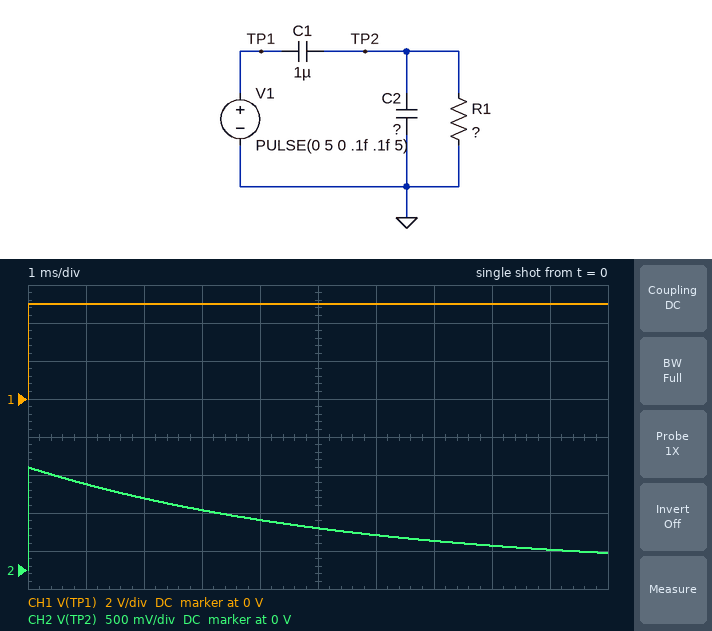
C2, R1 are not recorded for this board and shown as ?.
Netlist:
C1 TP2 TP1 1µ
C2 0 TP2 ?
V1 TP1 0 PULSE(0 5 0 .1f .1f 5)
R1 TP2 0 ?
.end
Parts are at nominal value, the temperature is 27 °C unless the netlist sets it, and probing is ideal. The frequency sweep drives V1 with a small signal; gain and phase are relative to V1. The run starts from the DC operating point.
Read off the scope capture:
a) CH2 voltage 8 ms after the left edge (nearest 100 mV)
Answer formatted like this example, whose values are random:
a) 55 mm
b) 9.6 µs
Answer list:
a) 300 mV
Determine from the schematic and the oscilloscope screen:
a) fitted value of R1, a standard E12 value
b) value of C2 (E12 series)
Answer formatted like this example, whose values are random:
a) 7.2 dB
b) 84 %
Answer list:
a) 1.5 kΩ
b) 2.7 µF
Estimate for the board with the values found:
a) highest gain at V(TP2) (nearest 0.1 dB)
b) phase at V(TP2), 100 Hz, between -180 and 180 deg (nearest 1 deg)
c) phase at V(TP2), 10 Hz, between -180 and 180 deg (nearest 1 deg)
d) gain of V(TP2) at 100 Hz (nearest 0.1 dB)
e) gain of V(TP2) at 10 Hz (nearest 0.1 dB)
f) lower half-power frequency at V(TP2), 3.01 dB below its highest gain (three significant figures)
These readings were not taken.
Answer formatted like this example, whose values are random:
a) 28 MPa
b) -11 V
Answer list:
a) -11.4 dB
b) 16 deg
c) 71 deg
d) -11.7 dB
e) -21.0 dB
f) 28.7 Hz
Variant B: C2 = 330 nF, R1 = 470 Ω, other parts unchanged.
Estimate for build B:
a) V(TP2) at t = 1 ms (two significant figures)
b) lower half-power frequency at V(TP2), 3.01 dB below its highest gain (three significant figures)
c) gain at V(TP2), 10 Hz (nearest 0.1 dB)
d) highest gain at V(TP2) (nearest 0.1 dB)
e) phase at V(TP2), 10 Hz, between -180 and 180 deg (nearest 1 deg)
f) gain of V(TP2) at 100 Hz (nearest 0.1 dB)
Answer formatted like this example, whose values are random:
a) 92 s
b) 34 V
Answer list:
a) 760 mV
b) 255 Hz
c) -30.6 dB
d) -2.5 dB
e) 88 deg
f) -11.2 dB
